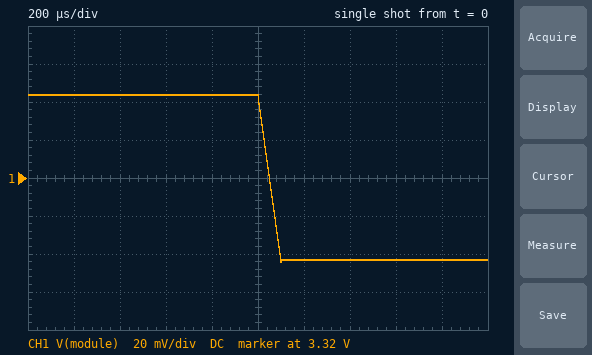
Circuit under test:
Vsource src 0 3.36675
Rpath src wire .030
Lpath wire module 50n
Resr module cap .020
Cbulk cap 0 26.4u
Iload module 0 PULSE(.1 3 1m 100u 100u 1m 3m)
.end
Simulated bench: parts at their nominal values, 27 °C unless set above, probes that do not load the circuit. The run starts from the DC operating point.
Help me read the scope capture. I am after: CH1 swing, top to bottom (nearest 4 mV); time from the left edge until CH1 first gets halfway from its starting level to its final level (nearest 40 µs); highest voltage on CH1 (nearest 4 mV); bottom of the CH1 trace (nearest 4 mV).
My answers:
88 mV
1.04 ms
3.364 V
3.276 V
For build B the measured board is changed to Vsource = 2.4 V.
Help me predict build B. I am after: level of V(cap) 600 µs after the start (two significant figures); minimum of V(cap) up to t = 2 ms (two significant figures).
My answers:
2.4 V
2.3 V
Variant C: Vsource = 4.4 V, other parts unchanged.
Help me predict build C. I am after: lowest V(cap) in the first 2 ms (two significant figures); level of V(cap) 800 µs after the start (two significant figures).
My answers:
4.3 V
4.4 V
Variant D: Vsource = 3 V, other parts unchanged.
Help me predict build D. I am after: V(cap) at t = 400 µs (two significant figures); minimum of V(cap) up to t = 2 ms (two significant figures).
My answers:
3.0 V
2.9 V
